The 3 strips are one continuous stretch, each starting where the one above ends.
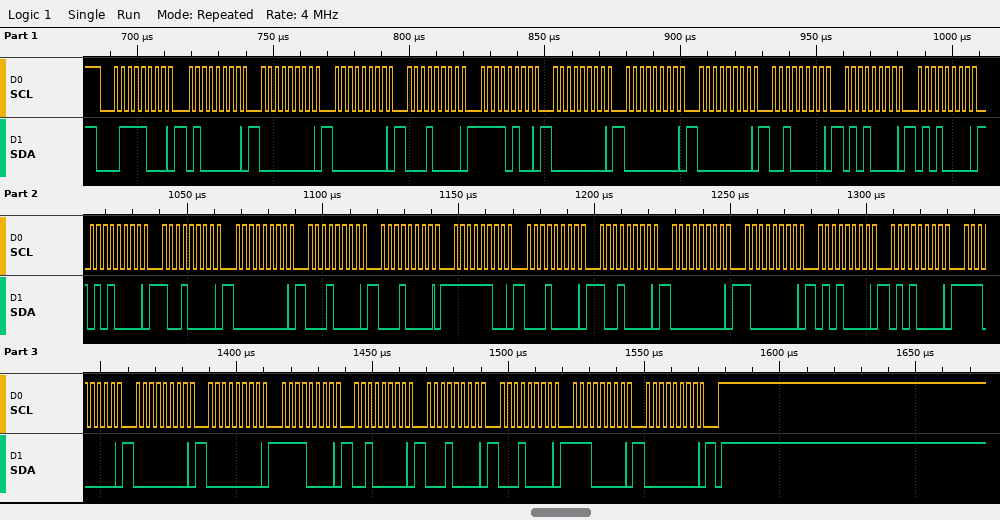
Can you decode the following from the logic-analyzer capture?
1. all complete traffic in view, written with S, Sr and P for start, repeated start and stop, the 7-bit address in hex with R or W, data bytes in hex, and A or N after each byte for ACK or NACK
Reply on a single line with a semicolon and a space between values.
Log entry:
S 3CW A 40 A 00 A 00 A 10 A F4 A 00 A 00 A 00 A 20 A 50 A 50 A 50 A 90 A 00 A 10 A 10 A FC A 10 A 90 A 00 A 80 A 50 A 50 A E0 A 00 A 00 A F0 A 20 A 10 A 10 A E0 A 00 A P
